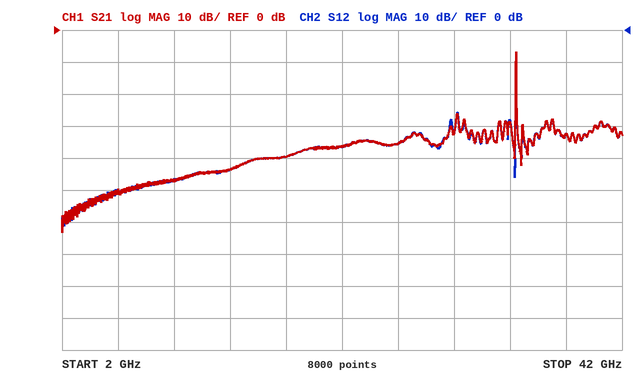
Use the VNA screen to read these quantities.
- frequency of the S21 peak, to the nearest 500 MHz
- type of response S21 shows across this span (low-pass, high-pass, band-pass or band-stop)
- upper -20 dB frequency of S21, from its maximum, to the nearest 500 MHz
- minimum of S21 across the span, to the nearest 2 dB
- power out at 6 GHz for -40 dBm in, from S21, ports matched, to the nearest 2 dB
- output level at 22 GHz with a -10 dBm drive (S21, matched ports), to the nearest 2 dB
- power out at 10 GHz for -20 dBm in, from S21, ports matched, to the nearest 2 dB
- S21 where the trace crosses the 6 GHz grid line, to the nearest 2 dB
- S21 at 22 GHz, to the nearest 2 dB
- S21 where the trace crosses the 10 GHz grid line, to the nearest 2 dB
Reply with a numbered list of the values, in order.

1. 34.5 GHz
2. band-pass
3. 34.5 GHz
4. -64 dB
5. -90 dBm
6. -46 dBm
7. -66 dBm
8. -50 dB
9. -36 dB
10. -46 dB
